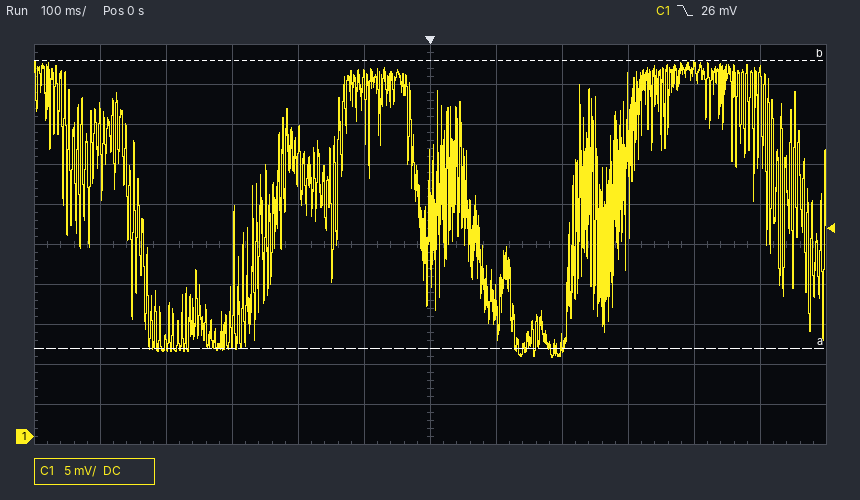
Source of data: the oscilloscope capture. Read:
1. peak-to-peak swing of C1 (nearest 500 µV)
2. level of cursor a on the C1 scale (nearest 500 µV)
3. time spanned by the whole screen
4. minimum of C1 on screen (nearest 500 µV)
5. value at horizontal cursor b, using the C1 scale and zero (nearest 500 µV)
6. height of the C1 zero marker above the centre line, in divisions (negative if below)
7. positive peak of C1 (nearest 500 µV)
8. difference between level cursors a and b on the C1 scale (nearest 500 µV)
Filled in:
37.0 mV
11.0 mV
1.2 s
10.0 mV
47.0 mV
-4.8 div
47.0 mV
36.0 mV
